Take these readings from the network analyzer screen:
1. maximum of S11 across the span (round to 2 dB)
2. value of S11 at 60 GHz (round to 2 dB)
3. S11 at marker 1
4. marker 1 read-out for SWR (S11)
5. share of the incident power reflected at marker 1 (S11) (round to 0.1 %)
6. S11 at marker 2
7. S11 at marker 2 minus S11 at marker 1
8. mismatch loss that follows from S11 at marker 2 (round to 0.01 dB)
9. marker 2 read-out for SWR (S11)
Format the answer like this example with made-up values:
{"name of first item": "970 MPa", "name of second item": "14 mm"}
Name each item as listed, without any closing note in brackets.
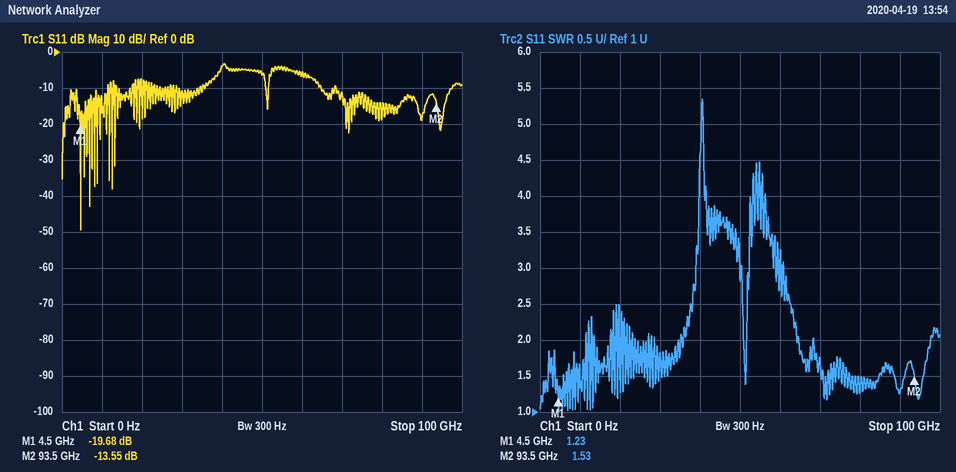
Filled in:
{"maximum of S11 across the span": "-4 dB", "value of S11 at 60 GHz": "-6 dB", "S11 at marker 1": "-19.68 dB", "marker 1 read-out for SWR": "1.23", "share of the incident power reflected at marker 1 (S11)": "1.1 %", "S11 at marker 2": "-13.55 dB", "S11 at marker 2 minus S11 at marker 1": "6.13 dB", "mismatch loss that follows from S11 at marker 2": "0.20 dB", "marker 2 read-out for SWR": "1.53"}
